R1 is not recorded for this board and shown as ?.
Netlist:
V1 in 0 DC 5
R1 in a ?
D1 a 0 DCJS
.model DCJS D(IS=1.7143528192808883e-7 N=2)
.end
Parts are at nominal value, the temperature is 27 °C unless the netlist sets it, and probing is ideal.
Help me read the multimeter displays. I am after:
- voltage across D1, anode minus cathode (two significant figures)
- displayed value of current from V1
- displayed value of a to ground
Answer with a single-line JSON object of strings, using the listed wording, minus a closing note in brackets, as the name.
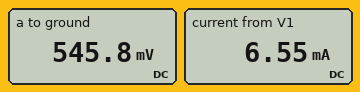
{"voltage across D1, anode minus cathode": "550 mV", "displayed value of current from V1": "6.55 mA", "displayed value of a to ground": "545.8 mV"}
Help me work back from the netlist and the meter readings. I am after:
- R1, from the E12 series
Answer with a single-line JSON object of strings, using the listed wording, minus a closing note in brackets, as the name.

{"R1, from the E12 series": "680 Ω"}
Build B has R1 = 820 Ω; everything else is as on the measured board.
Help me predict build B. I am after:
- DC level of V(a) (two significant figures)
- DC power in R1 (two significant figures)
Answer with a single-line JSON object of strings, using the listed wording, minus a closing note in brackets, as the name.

{"DC level of V(a)": "540 mV", "DC power in R1": "24 mW"}
